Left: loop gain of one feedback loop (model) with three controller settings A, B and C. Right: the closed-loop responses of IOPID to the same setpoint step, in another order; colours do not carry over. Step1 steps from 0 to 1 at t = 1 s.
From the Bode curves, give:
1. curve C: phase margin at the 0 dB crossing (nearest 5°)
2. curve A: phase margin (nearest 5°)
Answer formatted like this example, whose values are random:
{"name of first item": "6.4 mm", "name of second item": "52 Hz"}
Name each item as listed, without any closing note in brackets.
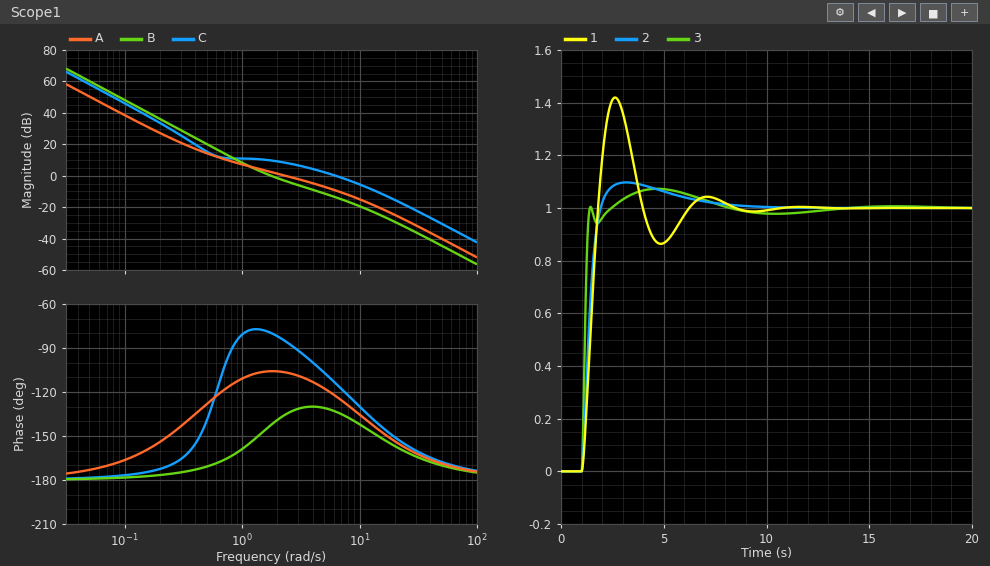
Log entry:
{"curve C: phase margin at the 0 dB crossing": "65°", "curve A: phase margin": "75°"}
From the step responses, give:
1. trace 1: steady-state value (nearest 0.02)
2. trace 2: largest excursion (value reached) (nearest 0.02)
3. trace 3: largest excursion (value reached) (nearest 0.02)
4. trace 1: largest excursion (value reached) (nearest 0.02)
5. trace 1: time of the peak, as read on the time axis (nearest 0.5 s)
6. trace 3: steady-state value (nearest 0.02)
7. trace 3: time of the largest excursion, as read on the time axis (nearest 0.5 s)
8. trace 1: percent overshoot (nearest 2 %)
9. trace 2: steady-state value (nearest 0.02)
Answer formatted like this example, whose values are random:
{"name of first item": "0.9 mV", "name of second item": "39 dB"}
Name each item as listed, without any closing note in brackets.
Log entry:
{"trace 1: steady-state value": "1.00", "trace 2: largest excursion (value reached)": "1.10", "trace 3: largest excursion (value reached)": "1.08", "trace 1: largest excursion (value reached)": "1.42", "trace 1: time of the peak, as read on the time axis": "2.5 s", "trace 3: steady-state value": "1.00", "trace 3: time of the largest excursion, as read on the time axis": "4.5 s", "trace 1: percent overshoot": "42 %", "trace 2: steady-state value": "1.00"}
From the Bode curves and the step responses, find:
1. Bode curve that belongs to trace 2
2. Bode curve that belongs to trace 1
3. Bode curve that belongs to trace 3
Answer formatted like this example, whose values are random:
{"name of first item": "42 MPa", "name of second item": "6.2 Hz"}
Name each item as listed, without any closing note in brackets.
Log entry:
{"Bode curve that belongs to trace 2": "A", "Bode curve that belongs to trace 1": "B", "Bode curve that belongs to trace 3": "C"}
